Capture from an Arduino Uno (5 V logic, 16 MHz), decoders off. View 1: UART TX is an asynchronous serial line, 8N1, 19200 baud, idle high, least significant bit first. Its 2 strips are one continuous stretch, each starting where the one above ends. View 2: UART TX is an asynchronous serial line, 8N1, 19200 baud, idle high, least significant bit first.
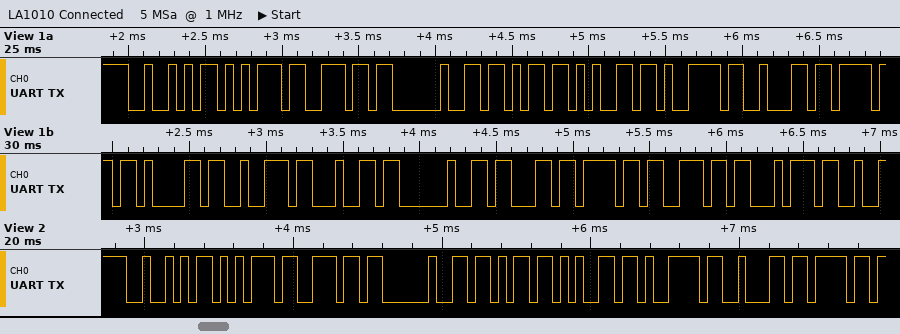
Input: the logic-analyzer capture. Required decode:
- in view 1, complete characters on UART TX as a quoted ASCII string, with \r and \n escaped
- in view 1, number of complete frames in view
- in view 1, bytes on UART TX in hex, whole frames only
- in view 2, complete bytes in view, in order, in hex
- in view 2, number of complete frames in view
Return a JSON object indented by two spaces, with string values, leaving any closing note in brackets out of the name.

{
  "in view 1, complete characters on UART TX as a quoted ASCII string, with \\r and \\n escaped": "\"Run keyboard cont\"",
  "in view 1, number of complete frames in view": "17",
  "in view 1, bytes on UART TX in hex, whole frames only": "52 75 6E 20 6B 65 79 62 6F 61 72 64 20 63 6F 6E 74",
  "in view 2, complete bytes in view, in order, in hex": "52 75 6E 20 6B 65 79 62 6F",
  "in view 2, number of complete frames in view": "9"
}
